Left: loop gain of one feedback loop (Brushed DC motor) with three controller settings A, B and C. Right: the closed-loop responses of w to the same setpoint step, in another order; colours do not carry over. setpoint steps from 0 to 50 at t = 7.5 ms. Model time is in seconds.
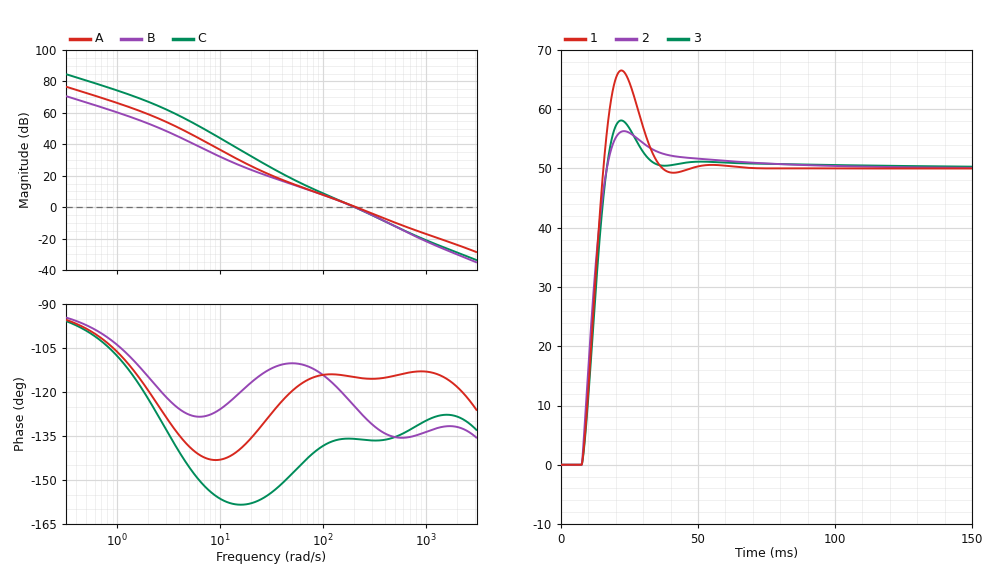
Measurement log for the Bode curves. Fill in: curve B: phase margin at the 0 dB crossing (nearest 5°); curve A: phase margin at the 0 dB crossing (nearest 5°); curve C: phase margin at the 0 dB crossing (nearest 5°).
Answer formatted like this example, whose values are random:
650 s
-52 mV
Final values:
55°
65°
45°
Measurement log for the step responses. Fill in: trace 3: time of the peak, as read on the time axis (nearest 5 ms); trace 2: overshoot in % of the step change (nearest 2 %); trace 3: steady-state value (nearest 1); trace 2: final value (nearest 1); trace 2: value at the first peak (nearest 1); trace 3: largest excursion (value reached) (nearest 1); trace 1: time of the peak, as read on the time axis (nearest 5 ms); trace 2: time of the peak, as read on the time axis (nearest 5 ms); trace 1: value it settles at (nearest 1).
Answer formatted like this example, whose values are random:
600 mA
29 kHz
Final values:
20 ms
12 %
50
50
56
58
20 ms
25 ms
50
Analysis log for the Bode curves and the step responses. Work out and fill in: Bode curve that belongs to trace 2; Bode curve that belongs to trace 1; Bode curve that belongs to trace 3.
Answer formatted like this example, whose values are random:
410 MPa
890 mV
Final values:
A
C
B
